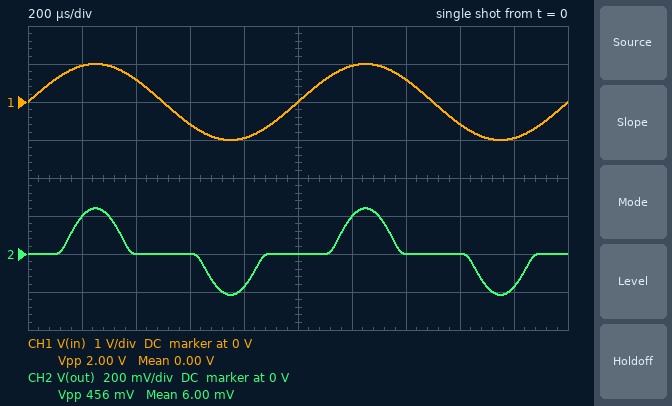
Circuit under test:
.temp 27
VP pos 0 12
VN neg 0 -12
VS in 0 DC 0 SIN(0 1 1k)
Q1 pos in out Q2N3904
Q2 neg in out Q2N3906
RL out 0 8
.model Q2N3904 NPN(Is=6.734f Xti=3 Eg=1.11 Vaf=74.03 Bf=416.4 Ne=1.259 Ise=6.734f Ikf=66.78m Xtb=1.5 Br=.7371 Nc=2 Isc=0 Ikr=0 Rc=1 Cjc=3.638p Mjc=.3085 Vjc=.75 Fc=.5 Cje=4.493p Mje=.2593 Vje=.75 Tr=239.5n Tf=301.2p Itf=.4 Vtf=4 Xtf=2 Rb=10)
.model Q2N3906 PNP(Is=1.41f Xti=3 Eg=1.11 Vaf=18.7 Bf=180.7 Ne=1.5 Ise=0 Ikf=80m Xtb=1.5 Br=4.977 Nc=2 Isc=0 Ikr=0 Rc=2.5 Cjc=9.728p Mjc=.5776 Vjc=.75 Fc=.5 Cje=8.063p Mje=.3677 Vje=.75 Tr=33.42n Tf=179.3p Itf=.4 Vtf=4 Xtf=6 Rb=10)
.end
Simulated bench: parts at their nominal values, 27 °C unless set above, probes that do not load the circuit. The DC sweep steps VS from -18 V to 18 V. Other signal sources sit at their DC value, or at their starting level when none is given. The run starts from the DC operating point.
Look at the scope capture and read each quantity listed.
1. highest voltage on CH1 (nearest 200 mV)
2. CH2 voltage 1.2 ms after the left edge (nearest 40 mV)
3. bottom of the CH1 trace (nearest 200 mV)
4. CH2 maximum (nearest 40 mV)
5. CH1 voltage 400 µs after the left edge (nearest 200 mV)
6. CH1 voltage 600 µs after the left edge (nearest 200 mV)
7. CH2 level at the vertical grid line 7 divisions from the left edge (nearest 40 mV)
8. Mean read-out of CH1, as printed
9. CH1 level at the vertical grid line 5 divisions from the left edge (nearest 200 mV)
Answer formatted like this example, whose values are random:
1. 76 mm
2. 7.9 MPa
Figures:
1. 1.0 V
2. 200 mV
3. -1.0 V
4. 240 mV
5. 600 mV
6. -600 mV
7. 0 V
8. 0.00 V
9. 0 V
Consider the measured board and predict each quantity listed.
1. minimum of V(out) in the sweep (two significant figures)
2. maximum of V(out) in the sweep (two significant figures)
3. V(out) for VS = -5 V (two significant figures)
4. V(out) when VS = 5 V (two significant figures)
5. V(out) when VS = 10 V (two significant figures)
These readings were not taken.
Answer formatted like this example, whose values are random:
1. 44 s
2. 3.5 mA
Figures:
1. -10 V
2. 11 V
3. -4.0 V
4. 4.0 V
5. 8.6 V
